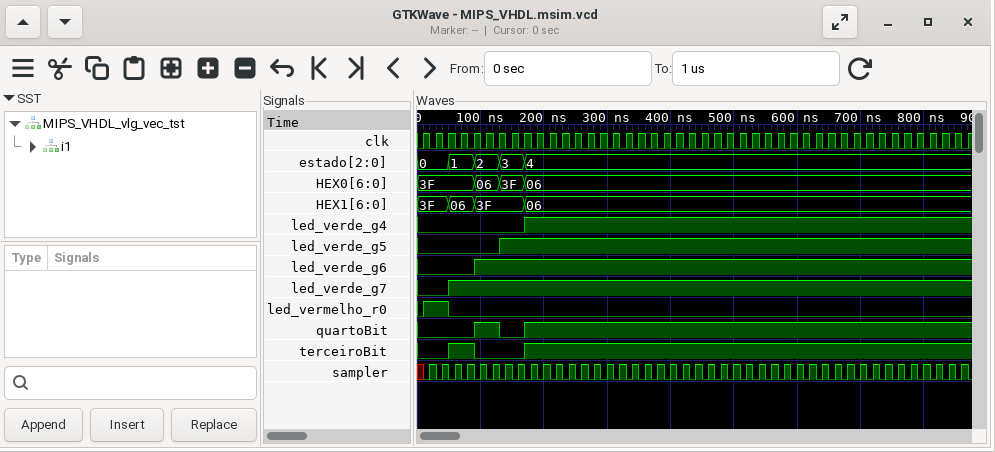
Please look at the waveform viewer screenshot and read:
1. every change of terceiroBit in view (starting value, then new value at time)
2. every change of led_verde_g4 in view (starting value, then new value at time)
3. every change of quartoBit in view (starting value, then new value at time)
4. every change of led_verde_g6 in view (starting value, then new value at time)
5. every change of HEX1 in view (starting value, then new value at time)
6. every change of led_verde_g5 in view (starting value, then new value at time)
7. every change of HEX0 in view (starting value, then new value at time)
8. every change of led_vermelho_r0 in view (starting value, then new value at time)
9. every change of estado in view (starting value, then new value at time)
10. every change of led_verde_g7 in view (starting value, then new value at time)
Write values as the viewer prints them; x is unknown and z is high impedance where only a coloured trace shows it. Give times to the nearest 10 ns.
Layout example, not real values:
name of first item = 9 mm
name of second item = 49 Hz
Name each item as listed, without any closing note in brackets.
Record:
every change of terceiroBit in view = 0, 1 at 50 ns, 0 at 90 ns, 1 at 170 ns
every change of led_verde_g4 in view = 0, 1 at 170 ns
every change of quartoBit in view = 0, 1 at 90 ns, 0 at 130 ns, 1 at 170 ns
every change of led_verde_g6 in view = 0, 1 at 90 ns
every change of HEX1 in view = 3F, 06 at 50 ns, 3F at 90 ns, 06 at 170 ns
every change of led_verde_g5 in view = 0, 1 at 130 ns
every change of HEX0 in view = 3F, 06 at 90 ns, 3F at 130 ns, 06 at 170 ns
every change of led_vermelho_r0 in view = 0, 1 at 10 ns, 0 at 50 ns
every change of estado in view = 0, 1 at 50 ns, 2 at 90 ns, 3 at 130 ns, 4 at 170 ns
every change of led_verde_g7 in view = 0, 1 at 50 ns
